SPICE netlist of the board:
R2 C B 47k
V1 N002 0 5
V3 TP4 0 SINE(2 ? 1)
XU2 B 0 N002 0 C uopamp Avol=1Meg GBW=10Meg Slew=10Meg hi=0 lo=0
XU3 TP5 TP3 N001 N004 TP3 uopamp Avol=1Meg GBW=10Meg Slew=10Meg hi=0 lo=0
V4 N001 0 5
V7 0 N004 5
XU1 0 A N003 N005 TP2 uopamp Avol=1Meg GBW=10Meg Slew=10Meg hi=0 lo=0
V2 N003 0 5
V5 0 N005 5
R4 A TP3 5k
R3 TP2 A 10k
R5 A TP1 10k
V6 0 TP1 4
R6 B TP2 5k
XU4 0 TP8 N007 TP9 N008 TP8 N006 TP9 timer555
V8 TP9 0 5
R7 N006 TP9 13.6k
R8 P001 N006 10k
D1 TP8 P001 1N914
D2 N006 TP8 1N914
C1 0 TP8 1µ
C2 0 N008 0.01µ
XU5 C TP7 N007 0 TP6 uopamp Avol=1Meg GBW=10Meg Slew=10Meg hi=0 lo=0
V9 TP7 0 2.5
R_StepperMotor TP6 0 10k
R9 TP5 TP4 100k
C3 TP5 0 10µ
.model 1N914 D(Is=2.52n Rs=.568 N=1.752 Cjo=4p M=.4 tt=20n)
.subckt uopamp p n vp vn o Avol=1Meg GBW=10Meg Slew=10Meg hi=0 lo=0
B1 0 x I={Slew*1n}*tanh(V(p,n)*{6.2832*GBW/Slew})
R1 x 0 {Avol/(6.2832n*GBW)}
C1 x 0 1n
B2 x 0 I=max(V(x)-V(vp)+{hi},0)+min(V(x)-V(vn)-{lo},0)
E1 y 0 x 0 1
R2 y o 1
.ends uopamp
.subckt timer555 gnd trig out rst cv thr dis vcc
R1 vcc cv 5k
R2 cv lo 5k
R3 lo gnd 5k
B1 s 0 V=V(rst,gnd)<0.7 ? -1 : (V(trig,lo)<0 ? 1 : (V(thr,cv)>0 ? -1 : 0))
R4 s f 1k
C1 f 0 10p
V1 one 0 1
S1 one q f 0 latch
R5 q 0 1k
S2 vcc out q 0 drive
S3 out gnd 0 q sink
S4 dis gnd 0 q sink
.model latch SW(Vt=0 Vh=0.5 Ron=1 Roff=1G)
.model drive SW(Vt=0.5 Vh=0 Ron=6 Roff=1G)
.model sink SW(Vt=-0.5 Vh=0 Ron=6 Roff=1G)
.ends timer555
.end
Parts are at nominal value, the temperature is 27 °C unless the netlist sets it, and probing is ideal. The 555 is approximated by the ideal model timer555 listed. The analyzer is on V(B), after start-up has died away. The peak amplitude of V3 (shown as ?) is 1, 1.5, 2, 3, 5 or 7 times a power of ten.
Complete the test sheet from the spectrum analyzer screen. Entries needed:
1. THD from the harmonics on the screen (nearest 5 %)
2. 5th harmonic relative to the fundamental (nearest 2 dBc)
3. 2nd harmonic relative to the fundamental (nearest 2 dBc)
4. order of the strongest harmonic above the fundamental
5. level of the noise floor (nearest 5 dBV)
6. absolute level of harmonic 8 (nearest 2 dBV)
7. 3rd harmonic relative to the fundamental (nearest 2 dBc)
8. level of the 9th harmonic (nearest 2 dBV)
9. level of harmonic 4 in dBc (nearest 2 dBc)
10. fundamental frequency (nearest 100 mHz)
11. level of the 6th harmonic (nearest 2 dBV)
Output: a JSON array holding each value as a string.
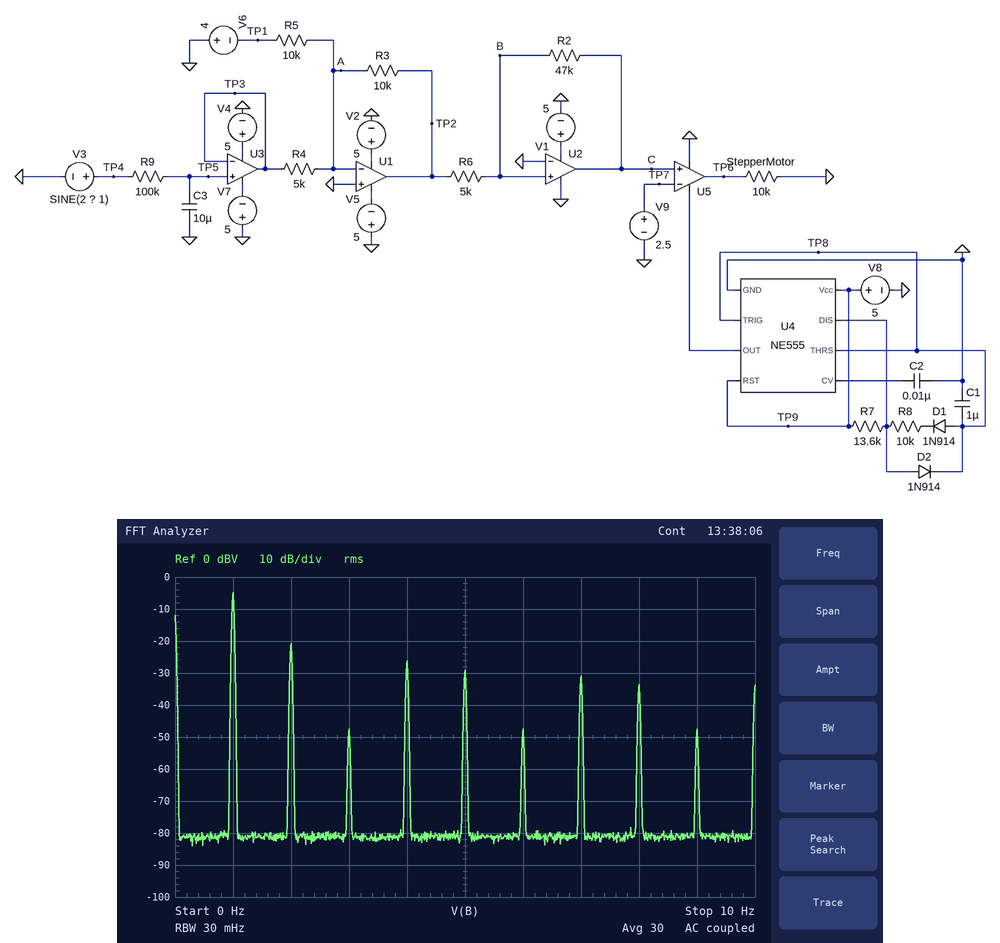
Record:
["20 %", "-24 dBc", "-16 dBc", "2", "-80 dBV", "-34 dBV", "-42 dBc", "-48 dBV", "-22 dBc", "1.0 Hz", "-48 dBV"]
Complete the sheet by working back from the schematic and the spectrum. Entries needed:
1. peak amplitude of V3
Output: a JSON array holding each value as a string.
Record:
["2 V"]
